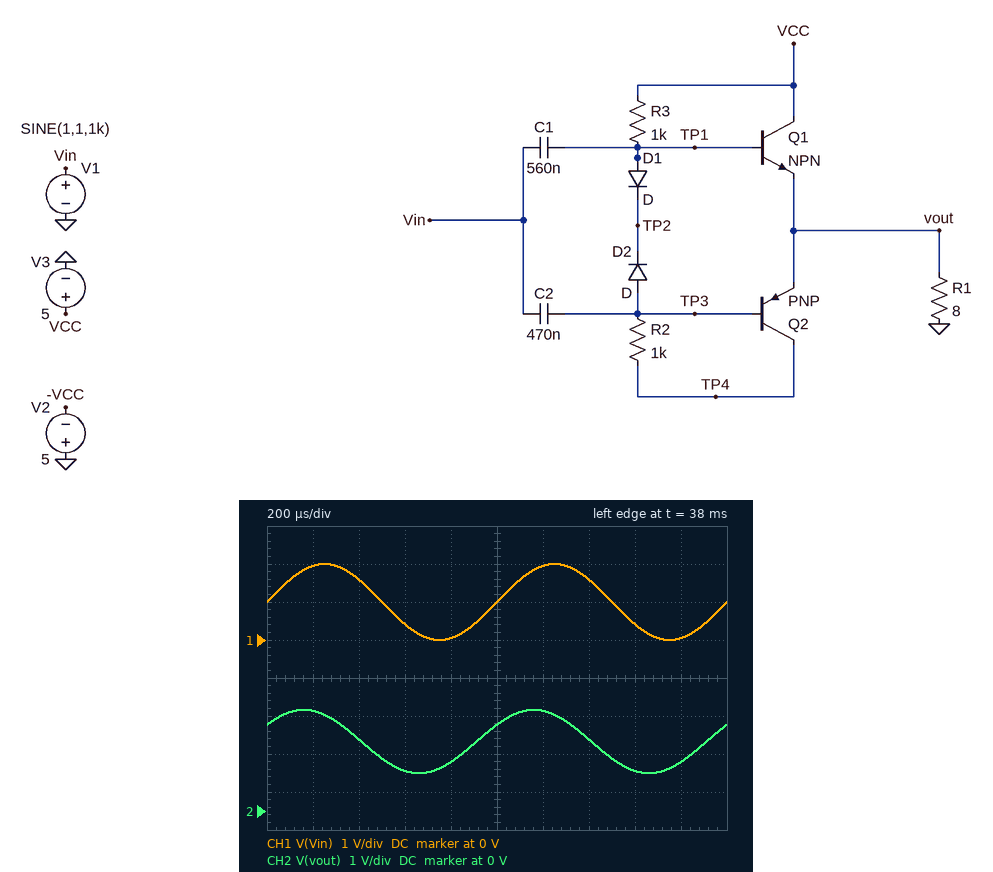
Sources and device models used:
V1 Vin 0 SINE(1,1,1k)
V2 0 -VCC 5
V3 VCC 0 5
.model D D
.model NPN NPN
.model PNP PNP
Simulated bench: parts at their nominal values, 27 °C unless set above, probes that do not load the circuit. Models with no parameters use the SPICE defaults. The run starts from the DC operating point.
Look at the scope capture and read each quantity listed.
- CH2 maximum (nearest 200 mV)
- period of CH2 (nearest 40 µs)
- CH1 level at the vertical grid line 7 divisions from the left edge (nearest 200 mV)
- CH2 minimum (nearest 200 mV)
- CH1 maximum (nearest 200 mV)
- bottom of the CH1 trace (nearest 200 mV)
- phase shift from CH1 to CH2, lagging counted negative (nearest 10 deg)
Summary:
2.6 V
1.00 ms
1.6 V
1.0 V
2.0 V
0 V
30 deg
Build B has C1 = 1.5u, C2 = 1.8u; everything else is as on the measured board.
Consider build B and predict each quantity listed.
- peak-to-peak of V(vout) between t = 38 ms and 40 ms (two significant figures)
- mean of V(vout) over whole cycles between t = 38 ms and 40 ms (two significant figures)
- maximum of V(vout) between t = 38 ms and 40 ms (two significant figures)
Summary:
1.9 V
1.8 V
2.8 V
